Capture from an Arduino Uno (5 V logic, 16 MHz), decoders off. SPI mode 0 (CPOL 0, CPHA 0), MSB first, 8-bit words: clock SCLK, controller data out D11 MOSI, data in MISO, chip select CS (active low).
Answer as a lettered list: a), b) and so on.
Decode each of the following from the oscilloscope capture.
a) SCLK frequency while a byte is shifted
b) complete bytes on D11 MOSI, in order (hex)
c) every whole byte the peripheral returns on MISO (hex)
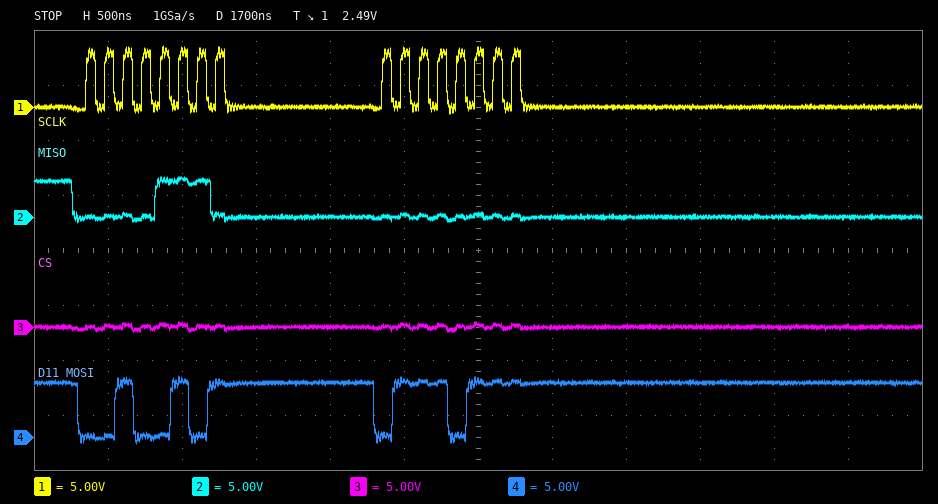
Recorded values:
a) 8 MHz
b) 25 77
c) 0E 00
